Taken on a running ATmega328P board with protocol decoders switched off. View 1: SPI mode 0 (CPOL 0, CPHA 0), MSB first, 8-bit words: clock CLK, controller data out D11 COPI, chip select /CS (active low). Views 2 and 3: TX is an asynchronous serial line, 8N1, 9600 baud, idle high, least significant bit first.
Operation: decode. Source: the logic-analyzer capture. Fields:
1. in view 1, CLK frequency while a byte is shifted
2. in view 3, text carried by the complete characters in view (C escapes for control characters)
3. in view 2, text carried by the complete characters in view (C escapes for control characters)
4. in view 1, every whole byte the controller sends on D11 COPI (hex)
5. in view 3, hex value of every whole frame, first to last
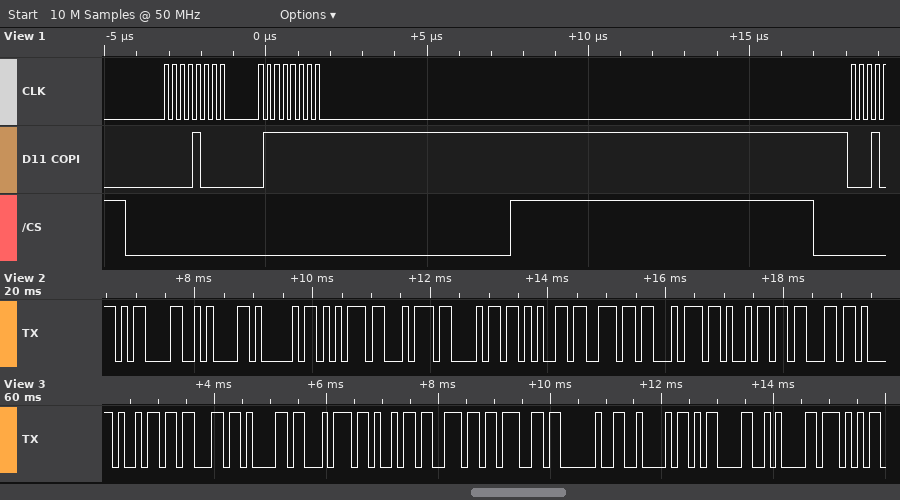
4 MHz
"icating B\r\nW"
"\r\nAuthentic"
08 7F
0x69 0x63 0x61 0x74 0x69 0x6E 0x67 0x20 0x42 0x0D 0x0A 0x57
